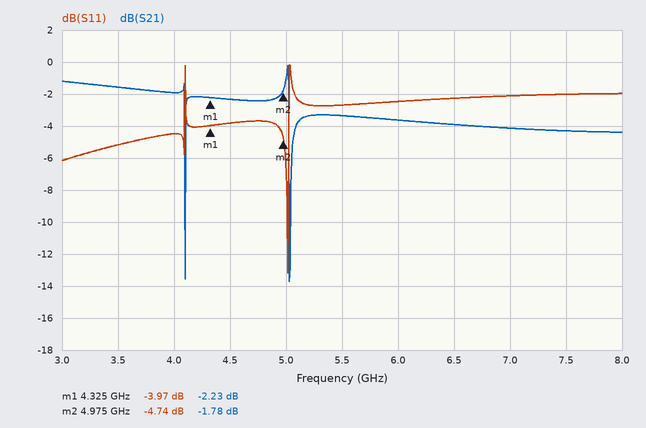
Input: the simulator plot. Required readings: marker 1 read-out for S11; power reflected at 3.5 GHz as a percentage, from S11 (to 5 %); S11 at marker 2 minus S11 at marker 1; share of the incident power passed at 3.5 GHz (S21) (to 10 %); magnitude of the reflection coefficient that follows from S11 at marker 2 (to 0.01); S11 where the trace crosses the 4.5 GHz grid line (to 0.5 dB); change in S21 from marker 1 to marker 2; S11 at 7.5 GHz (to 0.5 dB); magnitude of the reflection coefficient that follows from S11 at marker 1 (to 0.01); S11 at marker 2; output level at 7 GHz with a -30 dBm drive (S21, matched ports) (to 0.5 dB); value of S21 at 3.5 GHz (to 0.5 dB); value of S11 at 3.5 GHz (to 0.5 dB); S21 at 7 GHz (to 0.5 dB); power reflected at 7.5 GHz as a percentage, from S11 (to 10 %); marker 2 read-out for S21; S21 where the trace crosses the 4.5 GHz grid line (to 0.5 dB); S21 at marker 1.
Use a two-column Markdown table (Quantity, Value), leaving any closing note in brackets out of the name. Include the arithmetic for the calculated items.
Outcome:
| Quantity | Value |
|---|---|
| marker 1 read-out for S11 | -3.97 dB |
| power reflected at 3.5 GHz as a percentage, from S11 | 10^(-5/10) ≈ 31.6 %, so 30 % to the nearest 5 % |
| S11 at marker 2 minus S11 at marker 1 | -4.74 − (-3.97) = -0.77 dB |
| share of the incident power passed at 3.5 GHz (S21) | 10^(-1.5/10) ≈ 70.8 %, so 70 % to the nearest 10 % |
| magnitude of the reflection coefficient that follows from S11 at marker 2 | 10^(-4.74/20) ≈ 0.58 |
| S11 where the trace crosses the 4.5 GHz grid line | -4.0 dB |
| change in S21 from marker 1 to marker 2 | -1.78 − (-2.23) = 0.45 dB |
| S11 at 7.5 GHz | -2.0 dB |
| magnitude of the reflection coefficient that follows from S11 at marker 1 | 10^(-3.97/20) ≈ 0.63 |
| S11 at marker 2 | -4.74 dB |
| output level at 7 GHz with a -30 dBm drive (S21, matched ports) | -30 dBm + (-4.0 dB) = -34.0 dBm |
| value of S21 at 3.5 GHz | -1.5 dB |
| value of S11 at 3.5 GHz | -5.0 dB |
| S21 at 7 GHz | -4.0 dB |
| power reflected at 7.5 GHz as a percentage, from S11 | 10^(-2/10) ≈ 63.1 %, so 60 % to the nearest 10 % |
| marker 2 read-out for S21 | -1.78 dB |
| S21 where the trace crosses the 4.5 GHz grid line | -2.5 dB |
| S21 at marker 1 | -2.23 dB |
